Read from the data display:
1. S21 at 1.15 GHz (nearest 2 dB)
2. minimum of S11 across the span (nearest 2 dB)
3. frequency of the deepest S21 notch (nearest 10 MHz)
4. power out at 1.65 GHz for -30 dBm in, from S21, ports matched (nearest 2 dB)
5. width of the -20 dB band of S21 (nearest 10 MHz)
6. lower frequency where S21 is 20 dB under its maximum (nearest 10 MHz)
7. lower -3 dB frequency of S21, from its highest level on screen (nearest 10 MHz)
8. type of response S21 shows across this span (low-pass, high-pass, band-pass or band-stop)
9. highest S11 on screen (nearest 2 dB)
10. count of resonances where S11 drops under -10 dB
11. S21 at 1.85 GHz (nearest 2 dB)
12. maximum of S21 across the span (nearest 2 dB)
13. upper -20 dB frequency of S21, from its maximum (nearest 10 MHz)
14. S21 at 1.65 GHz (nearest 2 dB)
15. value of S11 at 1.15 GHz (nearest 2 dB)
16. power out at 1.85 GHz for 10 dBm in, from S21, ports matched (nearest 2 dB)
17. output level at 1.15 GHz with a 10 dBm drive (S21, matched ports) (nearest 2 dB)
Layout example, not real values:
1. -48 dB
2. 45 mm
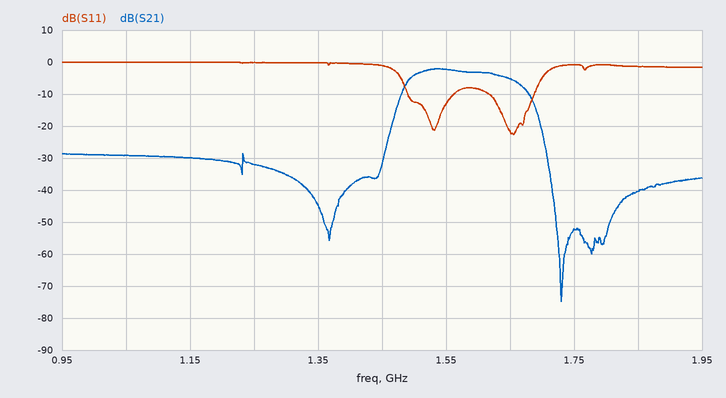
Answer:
1. -30 dB
2. -22 dB
3. 1.73 GHz
4. -36 dBm
5. 240 MHz
6. 1.46 GHz
7. 1.49 GHz
8. band-pass
9. 0 dB
10. 2
11. -40 dB
12. -2 dB
13. 1.70 GHz
14. -6 dB
15. 0 dB
16. -30 dBm
17. -20 dBm
